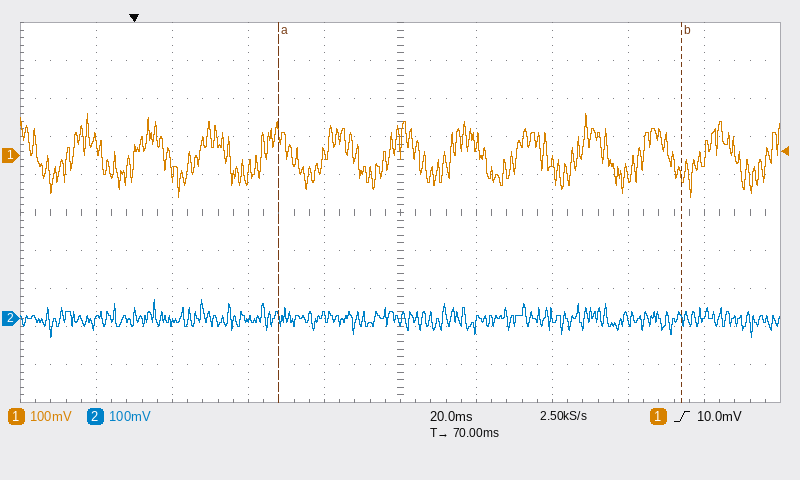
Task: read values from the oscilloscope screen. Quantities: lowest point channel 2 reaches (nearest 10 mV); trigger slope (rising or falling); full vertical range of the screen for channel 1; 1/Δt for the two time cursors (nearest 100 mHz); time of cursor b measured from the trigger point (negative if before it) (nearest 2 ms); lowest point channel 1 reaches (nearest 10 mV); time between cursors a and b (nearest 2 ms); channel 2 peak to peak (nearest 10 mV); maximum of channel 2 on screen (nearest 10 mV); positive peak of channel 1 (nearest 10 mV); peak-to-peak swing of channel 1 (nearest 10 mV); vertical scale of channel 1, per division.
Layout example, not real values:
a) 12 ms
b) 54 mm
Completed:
a) -50 mV
b) rising
c) 1 V
d) 9.4 Hz
e) +144 ms
f) -110 mV
g) 106 ms
h) 100 mV
i) 50 mV
j) 110 mV
k) 220 mV
l) 100 mV
